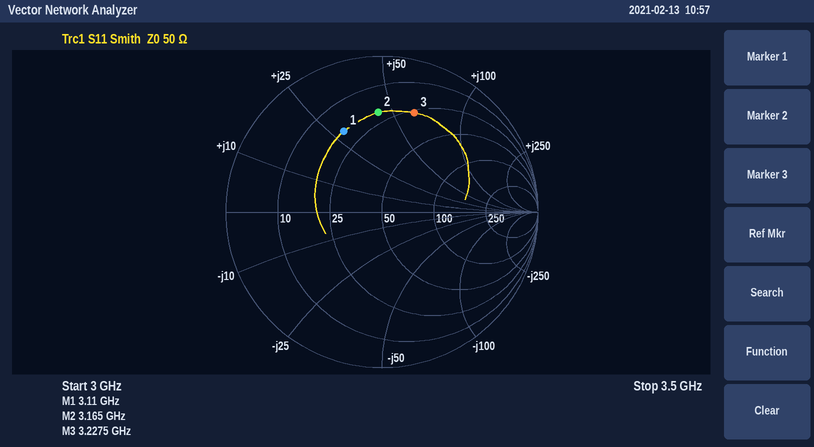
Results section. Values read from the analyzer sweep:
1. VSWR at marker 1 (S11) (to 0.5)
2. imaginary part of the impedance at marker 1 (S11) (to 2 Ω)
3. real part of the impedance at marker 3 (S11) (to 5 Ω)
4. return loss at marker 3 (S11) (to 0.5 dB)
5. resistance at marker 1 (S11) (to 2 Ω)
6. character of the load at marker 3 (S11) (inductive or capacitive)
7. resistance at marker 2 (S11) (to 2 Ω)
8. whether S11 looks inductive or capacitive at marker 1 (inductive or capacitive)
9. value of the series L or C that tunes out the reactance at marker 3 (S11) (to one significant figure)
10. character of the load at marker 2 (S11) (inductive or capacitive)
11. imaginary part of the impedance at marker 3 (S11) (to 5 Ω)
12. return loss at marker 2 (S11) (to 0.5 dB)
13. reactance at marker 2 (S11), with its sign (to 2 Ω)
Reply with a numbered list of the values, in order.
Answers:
1. 3.5
2. +28 Ω
3. 25 Ω
4. 3.5 dB
5. 18 Ω
6. inductive
7. 20 Ω
8. inductive
9. 800 fF
10. inductive
11. +60 Ω
12. 4.0 dB
13. +44 Ω
